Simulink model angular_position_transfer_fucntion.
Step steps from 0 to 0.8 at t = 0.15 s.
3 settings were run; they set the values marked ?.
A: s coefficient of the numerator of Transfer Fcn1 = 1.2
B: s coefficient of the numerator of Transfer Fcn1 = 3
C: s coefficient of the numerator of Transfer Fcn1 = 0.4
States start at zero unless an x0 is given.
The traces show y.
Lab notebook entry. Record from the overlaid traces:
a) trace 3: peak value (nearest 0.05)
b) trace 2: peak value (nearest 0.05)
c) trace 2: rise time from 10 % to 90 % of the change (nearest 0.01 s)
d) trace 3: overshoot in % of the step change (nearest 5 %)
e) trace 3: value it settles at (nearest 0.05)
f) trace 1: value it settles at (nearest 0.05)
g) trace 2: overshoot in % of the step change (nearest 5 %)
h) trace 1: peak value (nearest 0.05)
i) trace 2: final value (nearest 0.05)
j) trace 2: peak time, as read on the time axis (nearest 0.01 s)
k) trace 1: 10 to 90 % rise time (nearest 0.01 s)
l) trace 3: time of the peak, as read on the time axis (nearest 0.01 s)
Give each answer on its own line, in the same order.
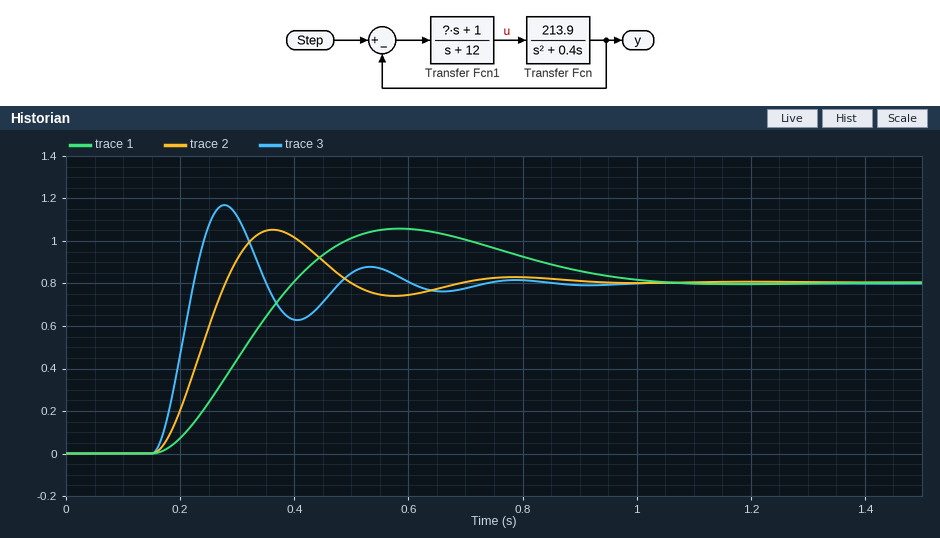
1.15
1.05
0.09 s
45 %
0.80
0.80
30 %
1.05
0.80
0.36 s
0.17 s
0.28 s
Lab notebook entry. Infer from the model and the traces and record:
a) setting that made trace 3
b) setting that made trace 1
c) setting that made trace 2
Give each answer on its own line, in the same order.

B
C
A
